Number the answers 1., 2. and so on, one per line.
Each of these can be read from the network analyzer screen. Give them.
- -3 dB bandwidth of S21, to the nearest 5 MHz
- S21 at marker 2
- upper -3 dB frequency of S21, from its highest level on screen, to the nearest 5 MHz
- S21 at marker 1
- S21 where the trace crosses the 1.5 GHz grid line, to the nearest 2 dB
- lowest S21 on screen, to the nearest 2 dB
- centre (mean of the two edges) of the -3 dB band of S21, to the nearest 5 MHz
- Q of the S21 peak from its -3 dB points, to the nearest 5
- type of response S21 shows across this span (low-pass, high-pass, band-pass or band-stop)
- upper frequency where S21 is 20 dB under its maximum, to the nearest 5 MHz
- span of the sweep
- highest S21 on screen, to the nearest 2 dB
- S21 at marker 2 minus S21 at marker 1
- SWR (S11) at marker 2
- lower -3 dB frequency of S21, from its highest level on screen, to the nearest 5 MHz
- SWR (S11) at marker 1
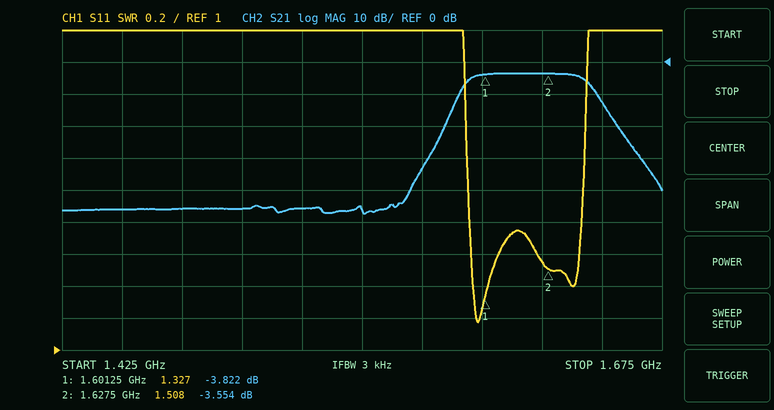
1. 50 MHz
2. -3.554 dB
3. 1.645 GHz
4. -3.822 dB
5. -46 dB
6. -48 dB
7. 1.620 GHz
8. 30
9. band-pass
10. 1.660 GHz
11. 250 MHz
12. -4 dB
13. 0.268 dB
14. 1.508
15. 1.595 GHz
16. 1.327
